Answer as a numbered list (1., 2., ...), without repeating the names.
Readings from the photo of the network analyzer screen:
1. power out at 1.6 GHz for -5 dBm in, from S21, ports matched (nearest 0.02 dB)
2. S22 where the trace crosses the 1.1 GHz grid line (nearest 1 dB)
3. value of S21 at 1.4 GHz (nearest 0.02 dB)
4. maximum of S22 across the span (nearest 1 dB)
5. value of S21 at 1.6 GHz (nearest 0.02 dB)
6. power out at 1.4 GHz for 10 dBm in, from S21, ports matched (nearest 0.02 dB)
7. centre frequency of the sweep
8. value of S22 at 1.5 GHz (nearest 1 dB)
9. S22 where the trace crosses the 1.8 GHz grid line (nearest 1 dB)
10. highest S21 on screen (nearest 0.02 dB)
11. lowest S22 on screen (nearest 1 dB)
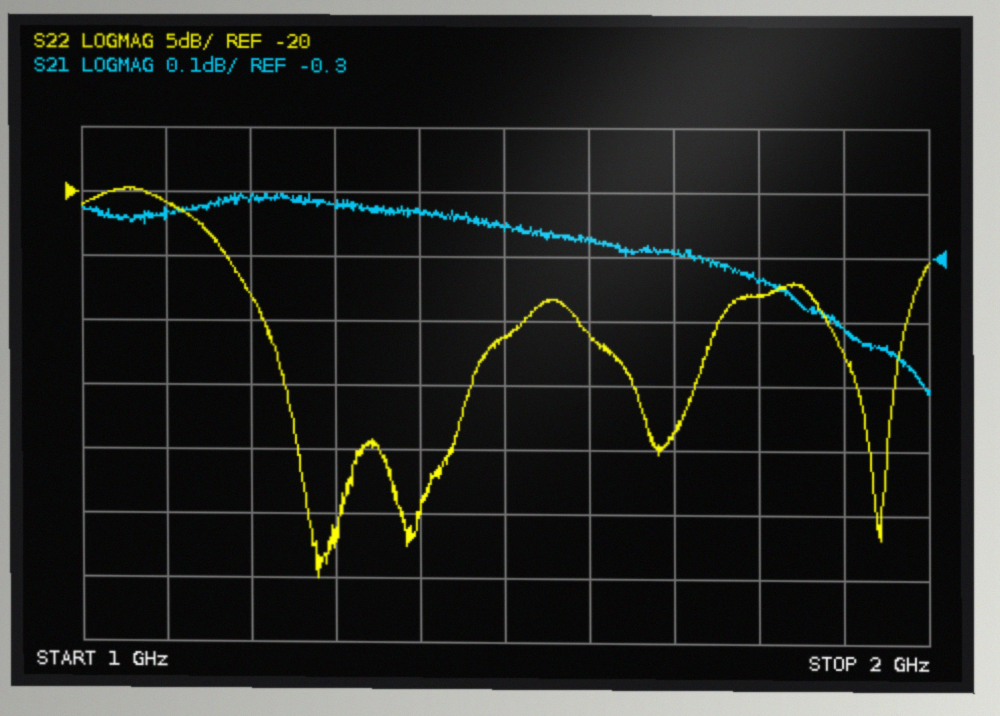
1. -5.28 dBm
2. -21 dB
3. -0.22 dB
4. -20 dB
5. -0.28 dB
6. 9.78 dBm
7. 1.5 GHz
8. -31 dB
9. -28 dB
10. -0.20 dB
11. -50 dB
